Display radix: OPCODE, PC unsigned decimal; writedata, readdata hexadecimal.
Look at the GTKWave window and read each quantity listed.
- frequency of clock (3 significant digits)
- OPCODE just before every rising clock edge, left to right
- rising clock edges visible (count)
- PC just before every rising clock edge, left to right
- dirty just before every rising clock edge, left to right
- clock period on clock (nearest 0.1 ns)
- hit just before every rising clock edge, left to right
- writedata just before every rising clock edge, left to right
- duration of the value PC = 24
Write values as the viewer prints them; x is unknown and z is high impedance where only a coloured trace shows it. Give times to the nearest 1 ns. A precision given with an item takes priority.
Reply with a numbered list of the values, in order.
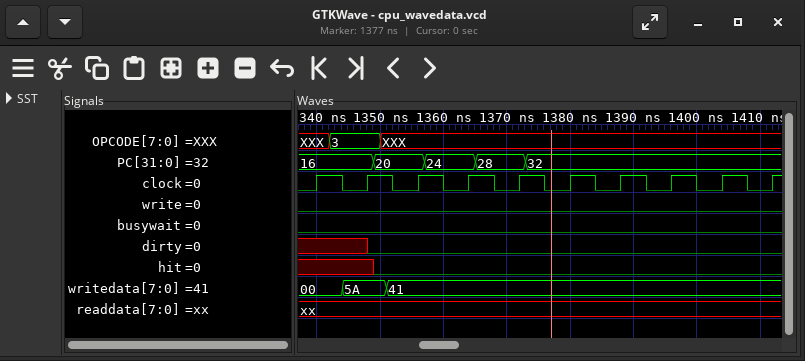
1. 125 MHz
2. XXX, 3, XXX, XXX, XXX, XXX, XXX, XXX, XXX, XXX
3. 10
4. 16, 16, 20, 24, 28, 32, 32, 32, 32, 32
5. x x 0 0 0 0 0 0 0 0
6. 8 ns
7. x x 0 0 0 0 0 0 0 0
8. 00, 5A, 41, 41, 41, 41, 41, 41, 41, 41
9. 8 ns
